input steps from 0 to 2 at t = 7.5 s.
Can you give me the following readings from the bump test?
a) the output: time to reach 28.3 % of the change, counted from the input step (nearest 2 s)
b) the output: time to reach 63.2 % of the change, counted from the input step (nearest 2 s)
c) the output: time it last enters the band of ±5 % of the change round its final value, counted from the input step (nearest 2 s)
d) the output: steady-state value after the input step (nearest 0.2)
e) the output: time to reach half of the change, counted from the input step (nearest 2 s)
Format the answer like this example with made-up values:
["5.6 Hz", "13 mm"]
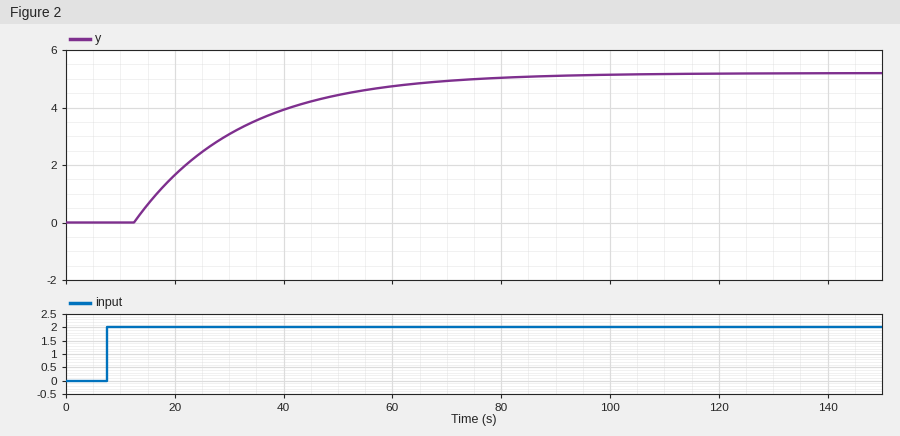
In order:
["12 s", "24 s", "64 s", "5.2", "18 s"]
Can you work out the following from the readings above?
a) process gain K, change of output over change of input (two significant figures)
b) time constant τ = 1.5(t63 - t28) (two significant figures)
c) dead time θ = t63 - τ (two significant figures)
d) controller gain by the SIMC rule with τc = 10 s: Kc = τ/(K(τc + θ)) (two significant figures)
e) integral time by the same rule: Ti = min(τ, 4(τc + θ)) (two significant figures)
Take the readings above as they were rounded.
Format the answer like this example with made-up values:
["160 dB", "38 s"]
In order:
["2.6", "18 s", "6.0 s", "0.43", "18 s"]
